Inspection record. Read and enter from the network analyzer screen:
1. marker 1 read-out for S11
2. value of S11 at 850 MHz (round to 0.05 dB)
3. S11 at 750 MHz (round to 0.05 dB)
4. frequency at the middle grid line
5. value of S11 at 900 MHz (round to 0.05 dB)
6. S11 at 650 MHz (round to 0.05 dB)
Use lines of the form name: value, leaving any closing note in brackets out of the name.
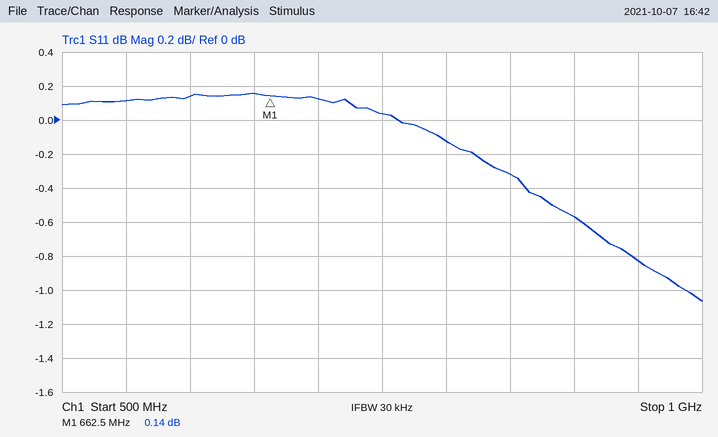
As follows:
marker 1 read-out for S11: 0.14 dB
value of S11 at 850 MHz: -0.30 dB
S11 at 750 MHz: 0.05 dB
frequency at the middle grid line: 750 MHz
value of S11 at 900 MHz: -0.55 dB
S11 at 650 MHz: 0.15 dB
